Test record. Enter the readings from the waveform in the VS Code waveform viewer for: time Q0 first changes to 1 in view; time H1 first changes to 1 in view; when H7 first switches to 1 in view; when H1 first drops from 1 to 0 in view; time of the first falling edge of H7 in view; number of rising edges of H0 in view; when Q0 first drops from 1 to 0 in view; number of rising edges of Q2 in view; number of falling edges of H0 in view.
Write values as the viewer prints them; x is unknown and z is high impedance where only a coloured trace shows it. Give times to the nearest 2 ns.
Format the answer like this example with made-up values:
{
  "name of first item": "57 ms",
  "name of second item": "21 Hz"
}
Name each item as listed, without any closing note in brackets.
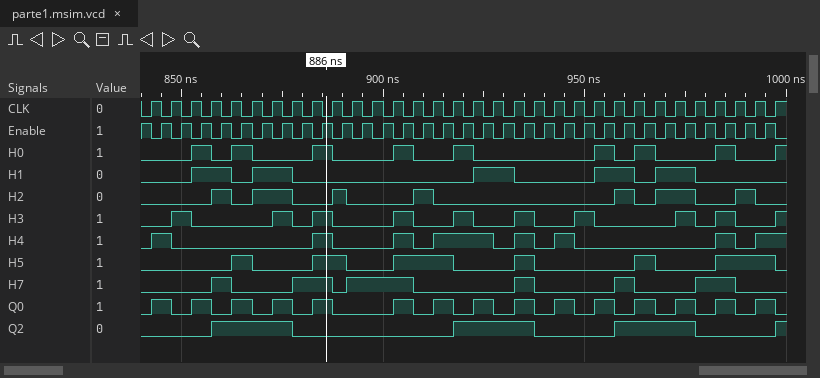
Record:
{
  "time Q0 first changes to 1 in view": "842 ns",
  "time H1 first changes to 1 in view": "852 ns",
  "when H7 first switches to 1 in view": "858 ns",
  "when H1 first drops from 1 to 0 in view": "862 ns",
  "time of the first falling edge of H7 in view": "862 ns",
  "number of rising edges of H0 in view": "9",
  "when Q0 first drops from 1 to 0 in view": "848 ns",
  "number of rising edges of Q2 in view": "4",
  "number of falling edges of H0 in view": "8"
}
